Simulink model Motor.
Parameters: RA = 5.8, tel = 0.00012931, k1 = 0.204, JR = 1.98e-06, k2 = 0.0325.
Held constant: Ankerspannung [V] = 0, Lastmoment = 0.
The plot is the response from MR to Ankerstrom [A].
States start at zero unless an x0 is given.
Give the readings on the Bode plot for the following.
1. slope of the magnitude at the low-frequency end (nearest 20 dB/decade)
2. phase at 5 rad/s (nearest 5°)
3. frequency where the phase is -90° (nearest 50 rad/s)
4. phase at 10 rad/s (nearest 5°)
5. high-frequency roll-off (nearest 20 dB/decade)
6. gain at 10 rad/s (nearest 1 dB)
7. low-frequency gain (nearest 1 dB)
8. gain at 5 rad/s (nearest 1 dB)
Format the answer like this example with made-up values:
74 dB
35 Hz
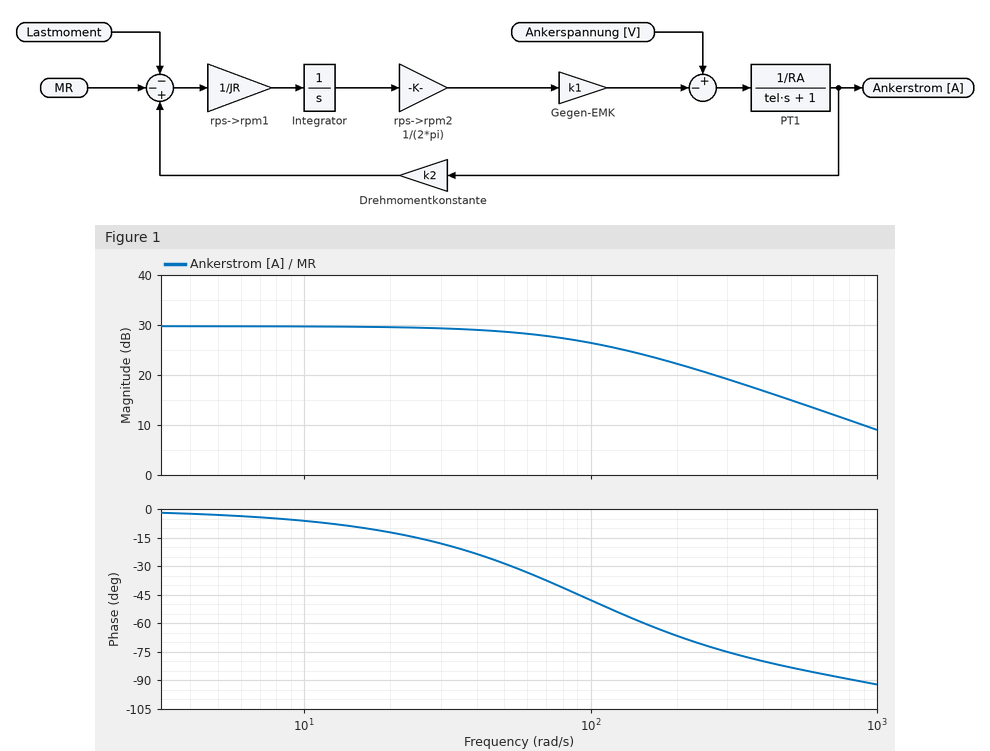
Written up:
0 dB/decade
-5°
850 rad/s
-5°
-20 dB/decade
30 dB
30 dB
30 dB
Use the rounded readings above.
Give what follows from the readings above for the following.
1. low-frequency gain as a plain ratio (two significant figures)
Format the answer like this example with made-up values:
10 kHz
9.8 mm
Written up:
32
